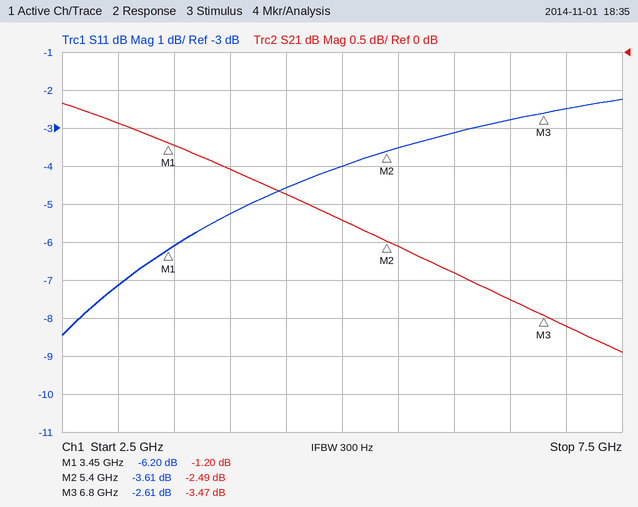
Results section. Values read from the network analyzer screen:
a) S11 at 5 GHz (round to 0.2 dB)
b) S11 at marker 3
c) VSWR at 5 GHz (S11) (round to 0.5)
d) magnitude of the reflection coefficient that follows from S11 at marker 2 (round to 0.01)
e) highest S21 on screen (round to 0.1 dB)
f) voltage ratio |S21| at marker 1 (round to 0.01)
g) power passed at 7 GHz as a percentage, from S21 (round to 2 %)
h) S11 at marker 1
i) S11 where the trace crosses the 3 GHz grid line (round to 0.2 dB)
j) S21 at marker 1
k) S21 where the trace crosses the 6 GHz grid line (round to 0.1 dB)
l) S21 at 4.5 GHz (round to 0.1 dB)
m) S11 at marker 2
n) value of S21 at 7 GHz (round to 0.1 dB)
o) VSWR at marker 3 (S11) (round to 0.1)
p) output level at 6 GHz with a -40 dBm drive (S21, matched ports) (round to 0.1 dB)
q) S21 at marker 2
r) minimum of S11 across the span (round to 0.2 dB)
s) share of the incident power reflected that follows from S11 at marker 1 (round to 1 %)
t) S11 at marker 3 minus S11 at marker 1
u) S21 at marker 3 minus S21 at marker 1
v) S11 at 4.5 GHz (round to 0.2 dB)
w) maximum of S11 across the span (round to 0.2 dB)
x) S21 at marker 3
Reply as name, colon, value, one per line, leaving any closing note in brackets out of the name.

S11 at 5 GHz: -4.0 dB
S11 at marker 3: -2.61 dB
VSWR at 5 GHz (S11): 4.5
magnitude of the reflection coefficient that follows from S11 at marker 2: 0.66
highest S21 on screen: -0.7 dB
voltage ratio |S21| at marker 1: 0.87
power passed at 7 GHz as a percentage, from S21: 44 %
S11 at marker 1: -6.20 dB
S11 where the trace crosses the 3 GHz grid line: -7.2 dB
S21 at marker 1: -1.20 dB
S21 where the trace crosses the 6 GHz grid line: -2.9 dB
S21 at 4.5 GHz: -1.9 dB
S11 at marker 2: -3.61 dB
value of S21 at 7 GHz: -3.6 dB
VSWR at marker 3 (S11): 6.7
output level at 6 GHz with a -40 dBm drive (S21, matched ports): -42.9 dBm
S21 at marker 2: -2.49 dB
minimum of S11 across the span: -8.4 dB
share of the incident power reflected that follows from S11 at marker 1: 24 %
S11 at marker 3 minus S11 at marker 1: 3.59 dB
S21 at marker 3 minus S21 at marker 1: -2.27 dB
S11 at 4.5 GHz: -4.6 dB
maximum of S11 across the span: -2.2 dB
S21 at marker 3: -3.47 dB
